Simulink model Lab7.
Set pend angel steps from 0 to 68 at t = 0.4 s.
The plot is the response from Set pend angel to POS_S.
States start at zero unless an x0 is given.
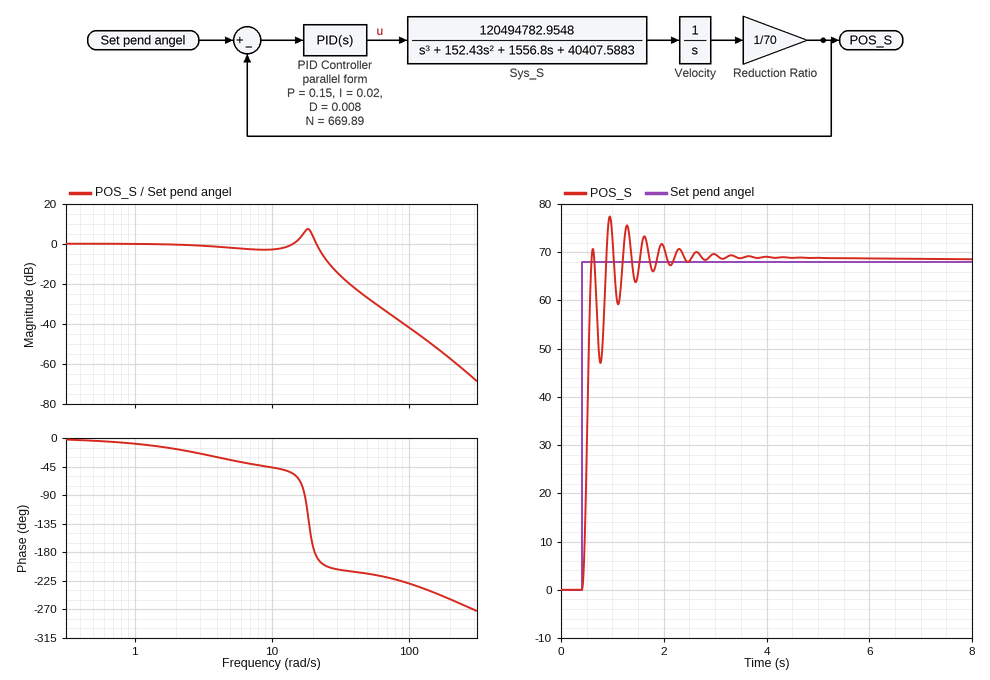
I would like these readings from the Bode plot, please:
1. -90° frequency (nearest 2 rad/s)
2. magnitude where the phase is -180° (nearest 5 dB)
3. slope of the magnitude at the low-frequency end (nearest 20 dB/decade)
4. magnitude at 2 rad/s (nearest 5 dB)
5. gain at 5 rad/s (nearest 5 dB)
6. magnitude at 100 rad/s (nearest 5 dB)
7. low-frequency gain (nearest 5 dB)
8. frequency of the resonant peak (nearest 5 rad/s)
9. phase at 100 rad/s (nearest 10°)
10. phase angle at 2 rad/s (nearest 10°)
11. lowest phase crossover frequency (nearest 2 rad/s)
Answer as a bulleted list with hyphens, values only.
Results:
- 18 rad/s
- 0 dB
- 0 dB/decade
- 0 dB
- 0 dB
- -40 dB
- 0 dB
- 20 rad/s
- -230°
- -20°
- 20 rad/s
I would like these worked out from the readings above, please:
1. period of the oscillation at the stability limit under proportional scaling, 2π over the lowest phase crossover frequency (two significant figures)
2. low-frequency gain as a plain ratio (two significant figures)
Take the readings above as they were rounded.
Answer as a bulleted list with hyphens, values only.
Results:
- 0.31 s
- 1.0
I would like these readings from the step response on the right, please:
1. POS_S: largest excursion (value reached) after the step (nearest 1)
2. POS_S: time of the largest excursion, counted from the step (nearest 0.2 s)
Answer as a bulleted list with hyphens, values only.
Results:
- 77
- 0.6 s
